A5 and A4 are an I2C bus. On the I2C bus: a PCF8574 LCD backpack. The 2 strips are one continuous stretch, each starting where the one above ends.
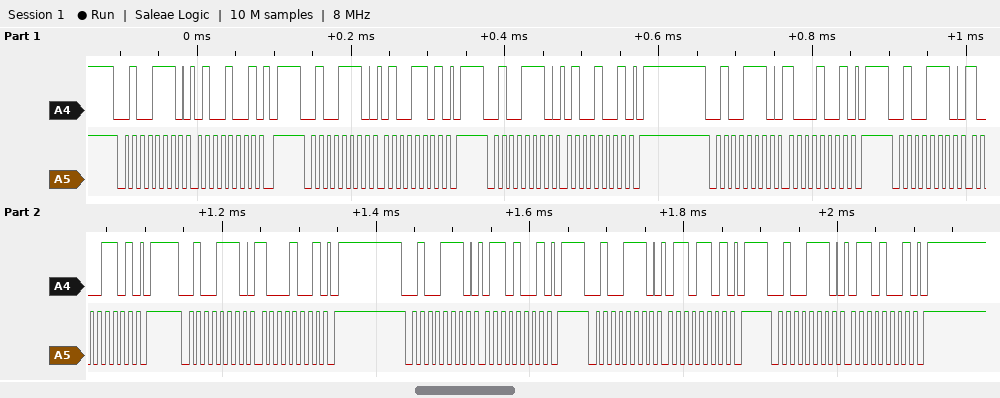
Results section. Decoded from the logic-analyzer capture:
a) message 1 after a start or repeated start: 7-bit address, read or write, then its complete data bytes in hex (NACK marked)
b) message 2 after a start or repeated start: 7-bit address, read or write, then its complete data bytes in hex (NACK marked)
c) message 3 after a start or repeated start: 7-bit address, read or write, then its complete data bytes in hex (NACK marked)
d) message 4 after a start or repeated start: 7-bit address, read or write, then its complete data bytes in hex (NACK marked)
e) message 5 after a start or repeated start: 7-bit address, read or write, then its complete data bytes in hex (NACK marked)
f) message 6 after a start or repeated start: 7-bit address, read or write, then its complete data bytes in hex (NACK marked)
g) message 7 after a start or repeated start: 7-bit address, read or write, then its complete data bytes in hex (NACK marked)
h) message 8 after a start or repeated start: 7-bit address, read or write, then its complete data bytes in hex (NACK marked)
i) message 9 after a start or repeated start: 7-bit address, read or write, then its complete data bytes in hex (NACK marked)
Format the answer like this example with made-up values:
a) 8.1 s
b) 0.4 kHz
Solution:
a) 0x27 write: 49
b) 0x27 write: 4D
c) 0x27 write: 49
d) 0x27 write: 89
e) 0x27 write: 8D
f) 0x27 write: 89
g) 0x27 write: 69
h) 0x27 write: 6D
i) 0x27 write: 69
